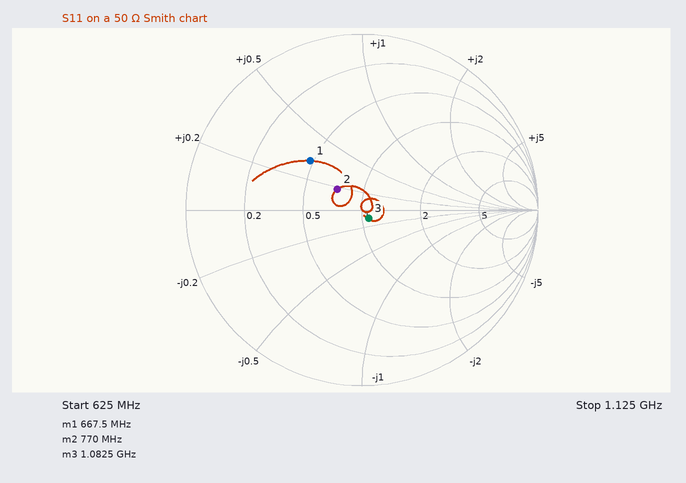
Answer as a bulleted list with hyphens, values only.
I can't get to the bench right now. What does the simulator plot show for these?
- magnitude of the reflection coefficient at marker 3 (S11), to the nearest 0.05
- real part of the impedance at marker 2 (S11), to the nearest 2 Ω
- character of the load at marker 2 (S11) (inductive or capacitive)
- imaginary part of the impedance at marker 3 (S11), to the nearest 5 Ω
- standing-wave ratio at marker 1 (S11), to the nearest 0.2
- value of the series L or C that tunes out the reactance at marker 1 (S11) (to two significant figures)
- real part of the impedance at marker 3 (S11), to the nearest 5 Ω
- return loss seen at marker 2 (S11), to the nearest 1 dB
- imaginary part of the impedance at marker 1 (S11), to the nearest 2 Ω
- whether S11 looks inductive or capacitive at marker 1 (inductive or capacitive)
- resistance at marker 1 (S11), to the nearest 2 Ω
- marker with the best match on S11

- 0.05
- 36 Ω
- inductive
- -5 Ω
- 2.4
- 15 pF
- 55 Ω
- 15 dB
- +16 Ω
- inductive
- 24 Ω
- marker 3
